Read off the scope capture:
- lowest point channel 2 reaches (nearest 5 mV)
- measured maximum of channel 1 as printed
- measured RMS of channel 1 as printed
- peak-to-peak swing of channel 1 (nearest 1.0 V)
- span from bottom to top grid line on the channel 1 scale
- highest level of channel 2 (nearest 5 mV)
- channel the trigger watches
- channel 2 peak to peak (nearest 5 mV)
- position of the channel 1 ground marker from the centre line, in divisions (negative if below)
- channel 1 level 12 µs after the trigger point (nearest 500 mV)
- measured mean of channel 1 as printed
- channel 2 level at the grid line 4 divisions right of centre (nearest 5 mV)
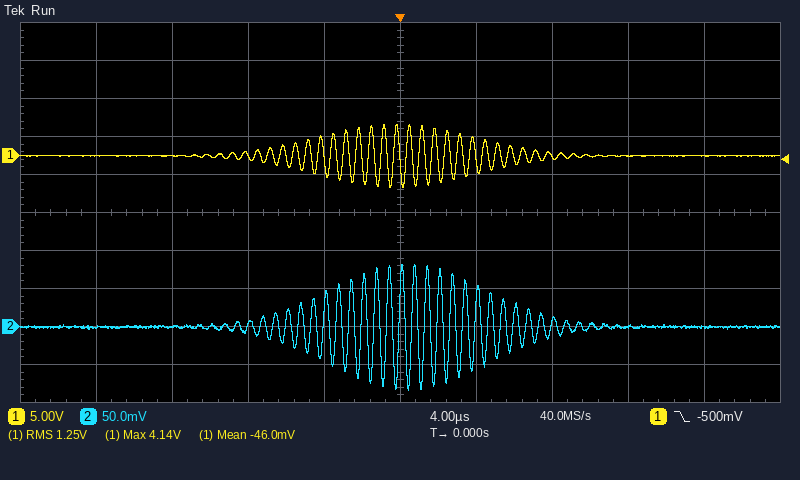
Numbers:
-85 mV
4.14 V
1.25 V
8.0 V
50 V
80 mV
channel 1
165 mV
+1.5 div
0.0 V
-46.0 mV
0 mV
